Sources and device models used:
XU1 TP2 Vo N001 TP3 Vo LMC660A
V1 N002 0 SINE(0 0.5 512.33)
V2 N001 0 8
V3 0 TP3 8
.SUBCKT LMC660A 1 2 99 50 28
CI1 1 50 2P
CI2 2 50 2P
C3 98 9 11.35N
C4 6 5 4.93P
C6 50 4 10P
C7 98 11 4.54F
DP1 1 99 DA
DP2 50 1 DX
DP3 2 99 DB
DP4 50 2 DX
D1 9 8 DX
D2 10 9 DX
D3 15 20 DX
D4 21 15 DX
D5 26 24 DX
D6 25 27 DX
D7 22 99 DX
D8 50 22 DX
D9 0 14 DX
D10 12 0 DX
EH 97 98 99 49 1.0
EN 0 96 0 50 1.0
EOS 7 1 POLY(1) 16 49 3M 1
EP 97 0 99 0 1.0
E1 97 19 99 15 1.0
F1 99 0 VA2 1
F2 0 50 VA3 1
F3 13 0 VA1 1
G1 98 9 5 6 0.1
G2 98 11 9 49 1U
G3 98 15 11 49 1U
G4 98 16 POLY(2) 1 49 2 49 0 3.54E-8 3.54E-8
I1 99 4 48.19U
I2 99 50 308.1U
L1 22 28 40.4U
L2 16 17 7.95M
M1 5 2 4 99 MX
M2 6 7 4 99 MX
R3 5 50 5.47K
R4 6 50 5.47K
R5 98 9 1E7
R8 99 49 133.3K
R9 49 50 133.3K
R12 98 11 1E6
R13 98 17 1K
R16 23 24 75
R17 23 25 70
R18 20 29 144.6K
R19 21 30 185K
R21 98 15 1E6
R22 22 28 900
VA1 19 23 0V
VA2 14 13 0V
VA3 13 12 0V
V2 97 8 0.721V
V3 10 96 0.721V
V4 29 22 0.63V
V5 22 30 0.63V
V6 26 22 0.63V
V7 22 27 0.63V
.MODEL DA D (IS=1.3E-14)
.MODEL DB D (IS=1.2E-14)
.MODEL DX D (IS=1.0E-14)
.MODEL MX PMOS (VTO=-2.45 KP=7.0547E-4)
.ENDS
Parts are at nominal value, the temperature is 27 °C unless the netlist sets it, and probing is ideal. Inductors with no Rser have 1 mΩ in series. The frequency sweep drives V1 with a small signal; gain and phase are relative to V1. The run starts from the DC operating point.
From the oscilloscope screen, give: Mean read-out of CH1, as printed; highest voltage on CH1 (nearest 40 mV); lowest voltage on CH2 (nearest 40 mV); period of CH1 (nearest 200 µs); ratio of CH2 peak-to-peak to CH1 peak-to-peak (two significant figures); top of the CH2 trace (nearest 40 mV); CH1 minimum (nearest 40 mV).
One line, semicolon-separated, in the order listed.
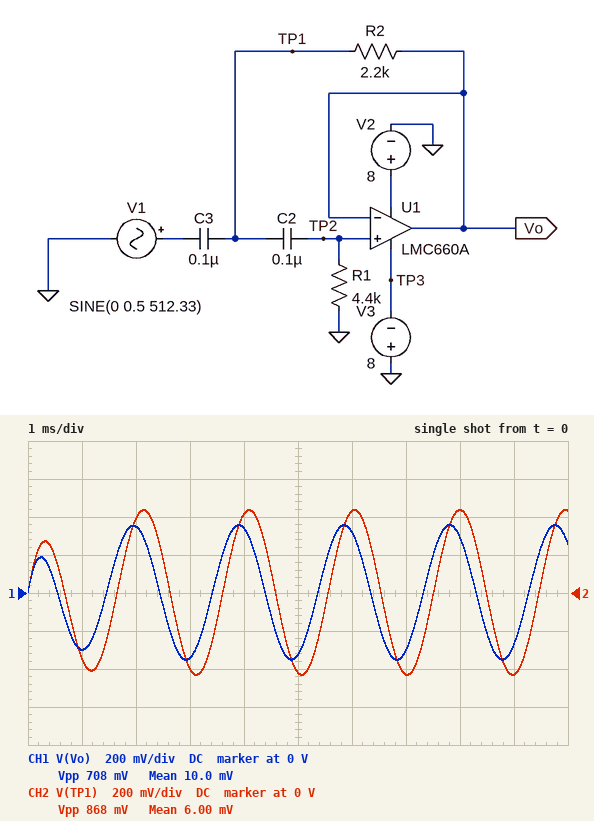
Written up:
10.0 mV; 360 mV; -440 mV; 2.0 ms; 1.2; 440 mV; -360 mV
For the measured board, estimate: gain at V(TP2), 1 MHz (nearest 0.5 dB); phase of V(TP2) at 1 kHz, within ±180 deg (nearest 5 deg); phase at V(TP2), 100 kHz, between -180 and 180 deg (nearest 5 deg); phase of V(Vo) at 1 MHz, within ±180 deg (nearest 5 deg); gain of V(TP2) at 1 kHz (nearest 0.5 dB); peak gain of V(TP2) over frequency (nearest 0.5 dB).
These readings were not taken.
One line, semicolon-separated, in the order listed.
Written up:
0 dB; 45 deg; 0 deg; -45 deg; -0.5 dB; 0 dB
